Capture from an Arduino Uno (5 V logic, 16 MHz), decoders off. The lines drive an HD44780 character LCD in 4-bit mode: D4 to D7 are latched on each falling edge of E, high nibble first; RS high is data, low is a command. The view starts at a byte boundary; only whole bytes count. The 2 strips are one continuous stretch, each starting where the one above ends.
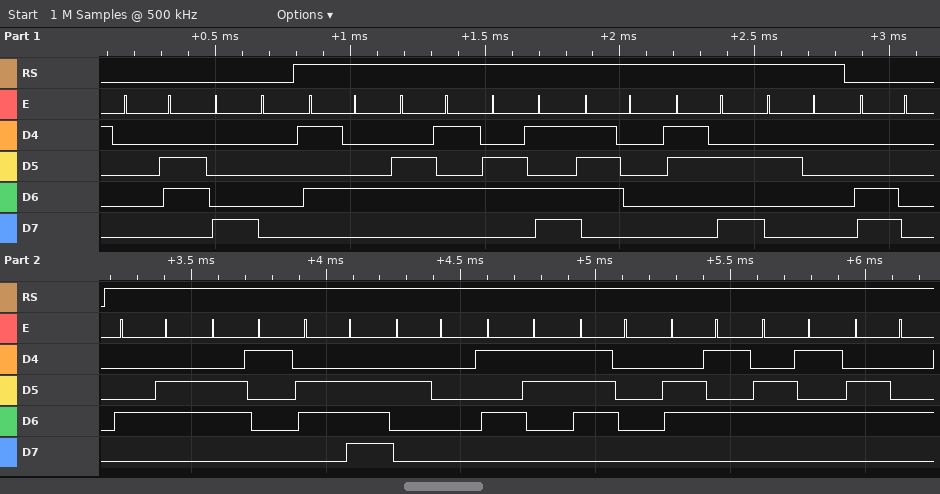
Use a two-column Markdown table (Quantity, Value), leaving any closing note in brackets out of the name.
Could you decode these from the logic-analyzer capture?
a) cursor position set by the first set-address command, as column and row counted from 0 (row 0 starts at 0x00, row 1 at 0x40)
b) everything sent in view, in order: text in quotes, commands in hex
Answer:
| Quantity | Value |
|---|---|
| cursor position set by the first set-address command, as column and row counted from 0 | column 0, row 0 |
| everything sent in view, in order: text in quotes, commands in hex | 0x06 0x80 "Temp: " 0xC0 "Fan Speed" |
